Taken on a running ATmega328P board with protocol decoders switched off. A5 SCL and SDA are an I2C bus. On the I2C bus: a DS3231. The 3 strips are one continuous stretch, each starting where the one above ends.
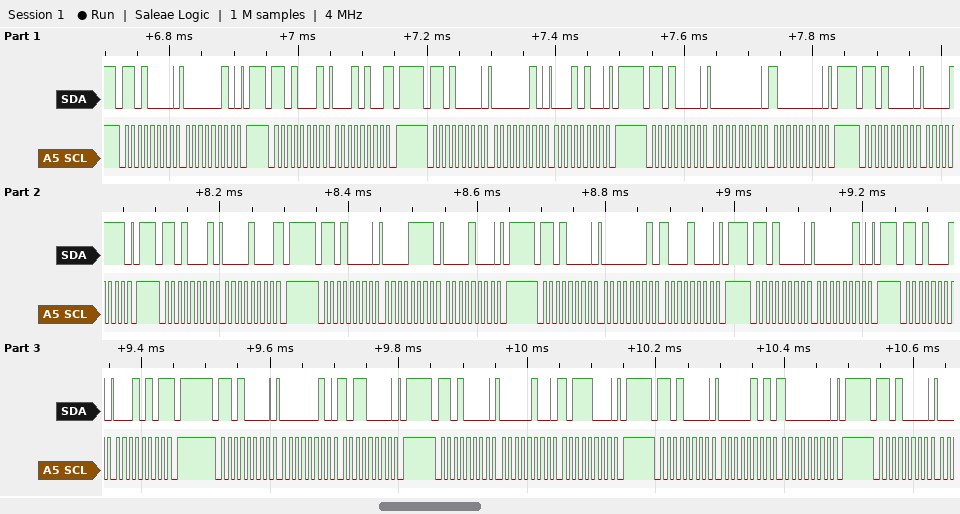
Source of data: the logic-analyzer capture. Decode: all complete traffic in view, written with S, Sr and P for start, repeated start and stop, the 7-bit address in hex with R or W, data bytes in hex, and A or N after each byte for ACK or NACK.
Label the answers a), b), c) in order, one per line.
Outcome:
a) S 68W A 02 A P S 68R A 14 N P S 68W A 02 A 14 A P S 68W A 00 A 80 A P S 68W A 0F A P S 68R A 08 N P S 68W A 0F A 08 A P S 68W A 01 A 88 A P S 68W A 02 A P S 68R A 15 N P S 68W A 02 A B0 A P S 68W A 04 A B8 A P S 68W A 05 A 80 A P S 68W A
